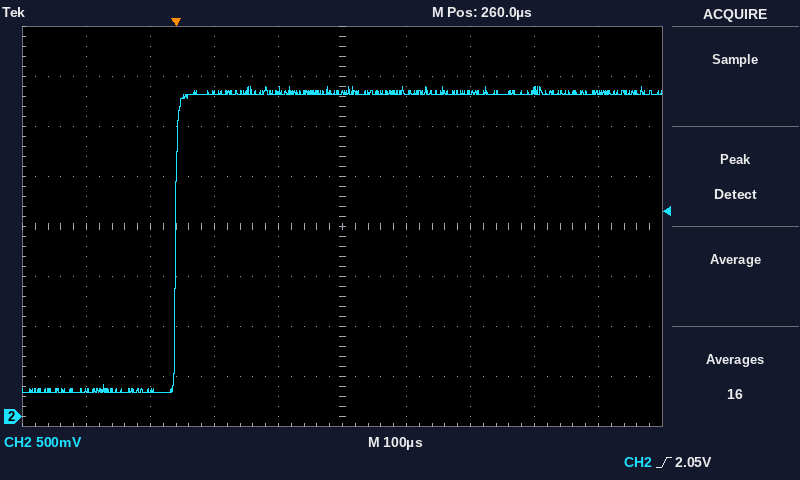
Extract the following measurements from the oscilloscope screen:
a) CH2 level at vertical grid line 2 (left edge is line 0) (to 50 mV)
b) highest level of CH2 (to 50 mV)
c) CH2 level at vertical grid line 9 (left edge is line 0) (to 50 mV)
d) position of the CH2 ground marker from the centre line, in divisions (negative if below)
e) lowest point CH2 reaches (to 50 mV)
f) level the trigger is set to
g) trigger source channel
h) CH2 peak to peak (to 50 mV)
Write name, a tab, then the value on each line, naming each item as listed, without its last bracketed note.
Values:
CH2 level at vertical grid line 2 (left edge is line 0)	250 mV
highest level of CH2	3.30 V
CH2 level at vertical grid line 9 (left edge is line 0)	3.25 V
position of the CH2 ground marker from the centre line, in divisions	-3.8 div
lowest point CH2 reaches	250 mV
level the trigger is set to	2.05 V
trigger source channel	CH2
CH2 peak to peak	3.05 V
